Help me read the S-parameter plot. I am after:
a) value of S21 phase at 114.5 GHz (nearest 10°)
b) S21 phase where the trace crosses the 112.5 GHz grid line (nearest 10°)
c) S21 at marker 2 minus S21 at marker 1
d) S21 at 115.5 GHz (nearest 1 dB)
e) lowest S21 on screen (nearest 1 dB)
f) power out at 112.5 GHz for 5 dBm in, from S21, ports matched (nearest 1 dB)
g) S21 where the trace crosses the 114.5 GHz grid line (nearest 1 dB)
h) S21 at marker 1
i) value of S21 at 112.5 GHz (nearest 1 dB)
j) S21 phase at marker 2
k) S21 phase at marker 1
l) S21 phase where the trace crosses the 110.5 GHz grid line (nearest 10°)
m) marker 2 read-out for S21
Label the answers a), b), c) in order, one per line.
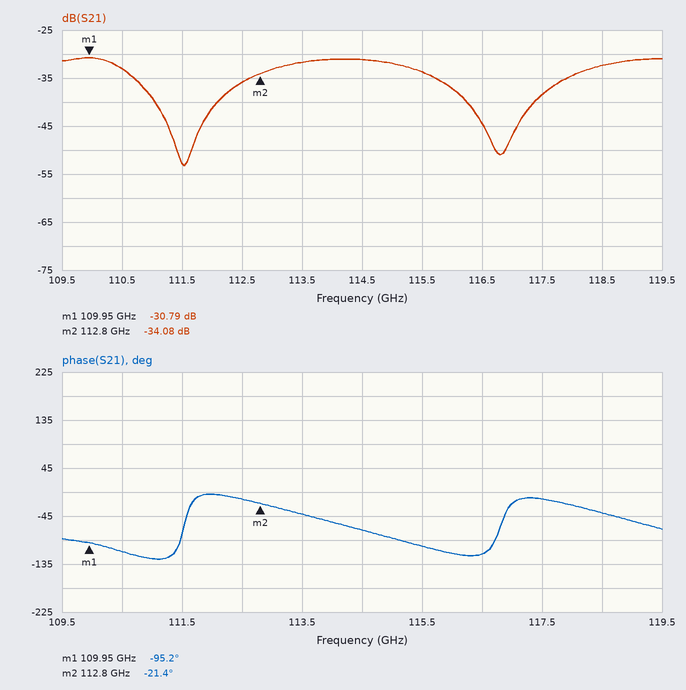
a) -70°
b) -10°
c) -3.29 dB
d) -34 dB
e) -53 dB
f) -31 dBm
g) -31 dB
h) -30.79 dB
i) -36 dB
j) -21.4°
k) -95.2°
l) -110°
m) -34.08 dB
